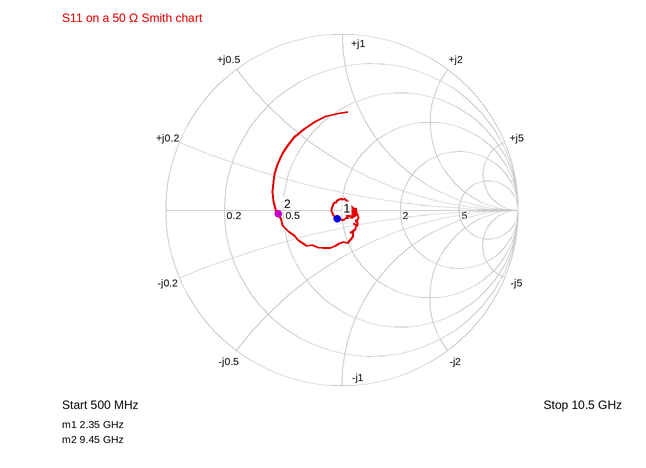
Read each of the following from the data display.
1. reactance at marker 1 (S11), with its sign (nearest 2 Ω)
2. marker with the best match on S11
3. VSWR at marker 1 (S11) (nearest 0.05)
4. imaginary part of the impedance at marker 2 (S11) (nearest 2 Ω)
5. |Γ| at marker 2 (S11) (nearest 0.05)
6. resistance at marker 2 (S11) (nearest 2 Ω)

-4 Ω
marker 1
1.10
-2 Ω
0.35
24 Ω
